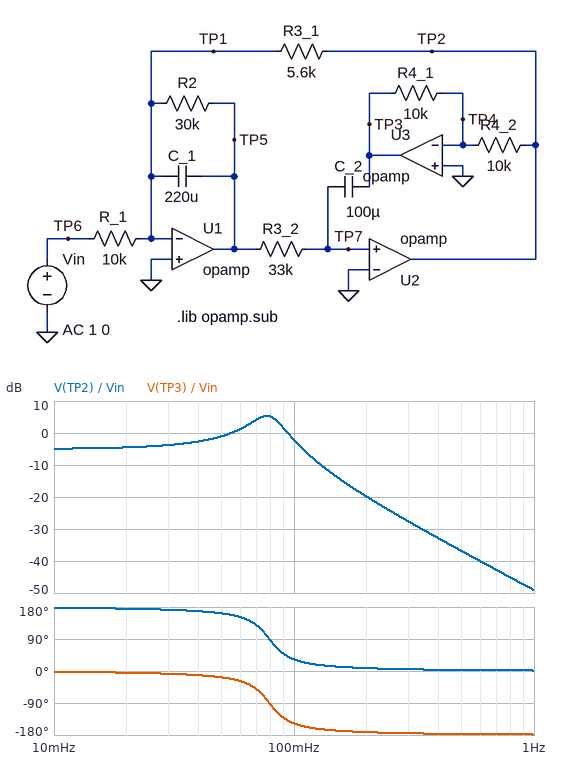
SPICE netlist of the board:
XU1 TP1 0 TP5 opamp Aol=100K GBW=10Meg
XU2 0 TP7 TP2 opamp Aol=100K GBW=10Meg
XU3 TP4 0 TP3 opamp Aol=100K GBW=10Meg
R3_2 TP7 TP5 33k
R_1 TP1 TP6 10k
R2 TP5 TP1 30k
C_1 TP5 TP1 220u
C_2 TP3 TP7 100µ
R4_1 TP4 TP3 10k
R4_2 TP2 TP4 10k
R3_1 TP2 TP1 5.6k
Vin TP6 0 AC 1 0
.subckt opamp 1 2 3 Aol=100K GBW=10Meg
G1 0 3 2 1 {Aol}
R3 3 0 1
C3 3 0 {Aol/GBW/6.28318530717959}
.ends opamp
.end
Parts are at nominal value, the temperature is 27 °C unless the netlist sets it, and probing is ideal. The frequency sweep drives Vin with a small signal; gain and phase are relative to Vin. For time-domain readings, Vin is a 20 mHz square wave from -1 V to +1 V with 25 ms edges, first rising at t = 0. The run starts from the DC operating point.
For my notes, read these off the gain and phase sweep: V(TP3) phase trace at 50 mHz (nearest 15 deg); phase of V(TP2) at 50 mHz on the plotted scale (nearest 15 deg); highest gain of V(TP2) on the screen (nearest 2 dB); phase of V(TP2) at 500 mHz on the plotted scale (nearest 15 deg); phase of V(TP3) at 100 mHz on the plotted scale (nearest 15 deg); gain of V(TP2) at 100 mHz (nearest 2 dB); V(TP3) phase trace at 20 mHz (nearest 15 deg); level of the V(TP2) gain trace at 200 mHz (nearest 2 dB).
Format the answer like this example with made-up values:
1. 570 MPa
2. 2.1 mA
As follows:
1. -15 deg
2. 165 deg
3. 6 dB
4. 0 deg
5. -150 deg
6. -2 dB
7. 0 deg
8. -20 dB
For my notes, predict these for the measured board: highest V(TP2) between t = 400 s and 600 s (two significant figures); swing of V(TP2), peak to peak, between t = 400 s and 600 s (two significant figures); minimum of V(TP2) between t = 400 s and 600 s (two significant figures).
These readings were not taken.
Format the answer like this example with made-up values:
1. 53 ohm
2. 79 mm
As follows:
1. 1.2 V
2. 2.3 V
3. -1.2 V
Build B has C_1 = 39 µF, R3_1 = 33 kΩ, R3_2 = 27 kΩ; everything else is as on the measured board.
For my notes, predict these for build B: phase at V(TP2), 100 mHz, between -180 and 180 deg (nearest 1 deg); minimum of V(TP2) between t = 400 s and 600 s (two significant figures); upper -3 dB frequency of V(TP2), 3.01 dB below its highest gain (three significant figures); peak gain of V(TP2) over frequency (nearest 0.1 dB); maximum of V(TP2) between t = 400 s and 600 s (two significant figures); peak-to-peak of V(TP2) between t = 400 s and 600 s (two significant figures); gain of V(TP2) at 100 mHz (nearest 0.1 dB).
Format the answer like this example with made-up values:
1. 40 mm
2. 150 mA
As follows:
1. 79 deg
2. -3.4 V
3. 74.7 mHz
4. 10.4 dB
5. 3.4 V
6. 6.8 V
7. 4.8 dB
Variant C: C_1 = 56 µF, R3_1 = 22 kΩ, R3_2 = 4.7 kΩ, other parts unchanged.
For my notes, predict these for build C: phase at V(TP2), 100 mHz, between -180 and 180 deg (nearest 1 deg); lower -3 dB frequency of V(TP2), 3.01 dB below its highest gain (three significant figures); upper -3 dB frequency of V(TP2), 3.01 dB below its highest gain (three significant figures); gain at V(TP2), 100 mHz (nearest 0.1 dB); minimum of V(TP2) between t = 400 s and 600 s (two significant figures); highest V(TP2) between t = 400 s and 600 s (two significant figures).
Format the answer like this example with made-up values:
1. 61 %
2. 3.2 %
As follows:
1. 164 deg
2. 141 mHz
3. 242 mHz
4. 8.8 dB
5. -4.3 V
6. 4.3 V
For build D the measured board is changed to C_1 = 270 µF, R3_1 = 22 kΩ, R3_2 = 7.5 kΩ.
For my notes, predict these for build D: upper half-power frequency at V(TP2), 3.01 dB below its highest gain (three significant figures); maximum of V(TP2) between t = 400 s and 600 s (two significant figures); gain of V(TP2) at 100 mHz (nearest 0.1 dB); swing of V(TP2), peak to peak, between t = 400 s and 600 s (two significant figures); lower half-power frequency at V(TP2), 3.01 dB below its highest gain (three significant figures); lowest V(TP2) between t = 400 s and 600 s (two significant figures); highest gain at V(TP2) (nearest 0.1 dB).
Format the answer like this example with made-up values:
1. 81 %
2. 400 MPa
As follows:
1. 83.4 mHz
2. 4.8 V
3. 8.4 dB
4. 9.5 V
5. 63.4 mHz
6. -4.8 V
7. 18.6 dB
